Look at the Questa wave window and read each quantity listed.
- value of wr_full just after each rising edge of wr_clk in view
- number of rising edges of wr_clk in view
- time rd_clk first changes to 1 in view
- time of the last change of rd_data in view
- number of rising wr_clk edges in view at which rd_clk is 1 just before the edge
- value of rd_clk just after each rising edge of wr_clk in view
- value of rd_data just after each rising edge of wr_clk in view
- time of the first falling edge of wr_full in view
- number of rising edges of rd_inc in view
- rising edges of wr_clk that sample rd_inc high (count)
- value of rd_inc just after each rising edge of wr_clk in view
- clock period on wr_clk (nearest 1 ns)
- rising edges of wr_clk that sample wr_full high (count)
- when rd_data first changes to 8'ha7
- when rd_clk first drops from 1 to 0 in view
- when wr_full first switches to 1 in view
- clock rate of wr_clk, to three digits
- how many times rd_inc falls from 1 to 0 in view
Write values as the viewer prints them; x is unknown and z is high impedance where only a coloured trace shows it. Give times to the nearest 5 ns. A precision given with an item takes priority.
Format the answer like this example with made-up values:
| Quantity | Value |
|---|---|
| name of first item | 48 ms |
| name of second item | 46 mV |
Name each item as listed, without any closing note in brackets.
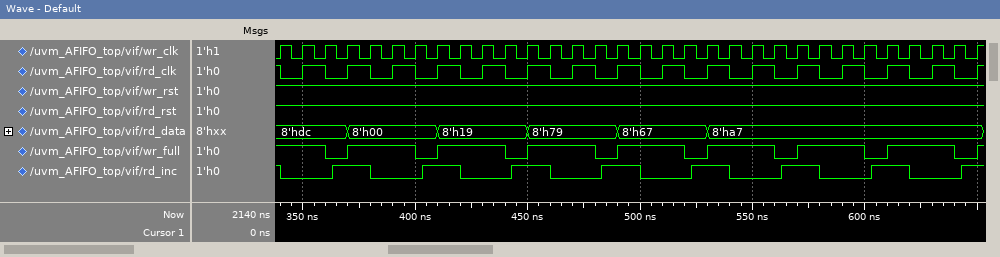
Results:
| Quantity | Value |
|---|---|
| value of wr_full just after each rising edge of wr_clk in view | 1 1 0 1 1 1 0 1 1 1 0 1 1 1 0 1 1 1 0 1 1 1 0 1 1 1 0 1 1 1 0 1 |
| number of rising edges of wr_clk in view | 32 |
| time rd_clk first changes to 1 in view | 350 ns |
| time of the last change of rd_data in view | 530 ns |
| number of rising wr_clk edges in view at which rd_clk is 1 just before the edge | 16 |
| value of rd_clk just after each rising edge of wr_clk in view | 0 1 0 1 0 1 0 1 0 1 0 1 0 1 0 1 0 1 0 1 0 1 0 1 0 1 0 1 0 1 0 1 |
| value of rd_data just after each rising edge of wr_clk in view | 8'hdc, 8'hdc, 8'hdc, 8'h00, 8'h00, 8'h00, 8'h00, 8'h19, 8'h19, 8'h19, 8'h19, 8'h79, 8'h79, 8'h79, 8'h79, 8'h67, 8'h67, 8'h67, 8'h67, 8'ha7, 8'ha7, 8'ha7, 8'ha7, 8'ha7, 8'ha7, 8'ha7, 8'ha7, 8'ha7, 8'ha7, 8'ha7, 8'ha7, 8'ha7 |
| time of the first falling edge of wr_full in view | 360 ns |
| number of rising edges of rd_inc in view | 8 |
| rising edges of wr_clk that sample rd_inc high | 16 |
| value of rd_inc just after each rising edge of wr_clk in view | 0 0 0 1 0 0 0 1 0 0 0 1 0 0 0 1 0 0 0 1 0 0 0 1 0 0 0 1 0 0 0 1 |
| clock period on wr_clk | 10 ns |
| rising edges of wr_clk that sample wr_full high | 24 |
| when rd_data first changes to 8'ha7 | 530 ns |
| when rd_clk first drops from 1 to 0 in view | 340 ns |
| when wr_full first switches to 1 in view | 370 ns |
| clock rate of wr_clk, to three digits | 100 MHz |
| how many times rd_inc falls from 1 to 0 in view | 8 |
